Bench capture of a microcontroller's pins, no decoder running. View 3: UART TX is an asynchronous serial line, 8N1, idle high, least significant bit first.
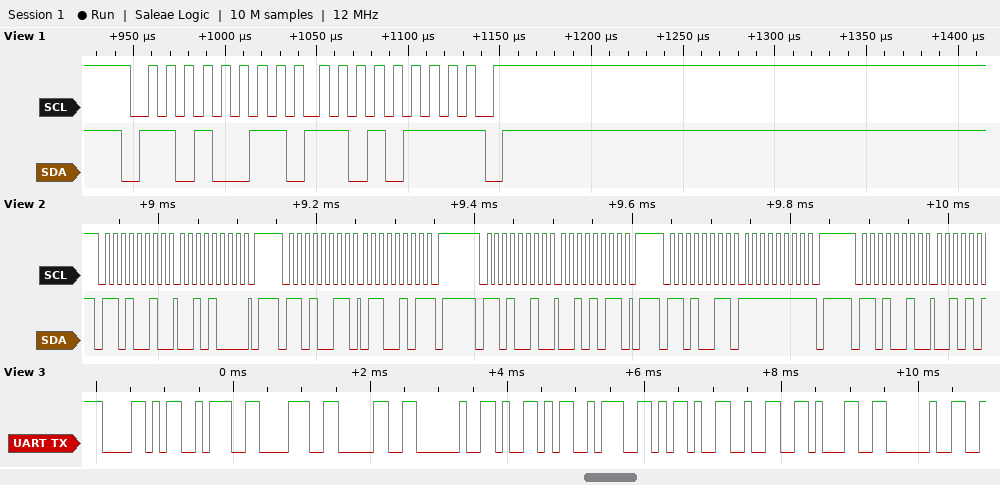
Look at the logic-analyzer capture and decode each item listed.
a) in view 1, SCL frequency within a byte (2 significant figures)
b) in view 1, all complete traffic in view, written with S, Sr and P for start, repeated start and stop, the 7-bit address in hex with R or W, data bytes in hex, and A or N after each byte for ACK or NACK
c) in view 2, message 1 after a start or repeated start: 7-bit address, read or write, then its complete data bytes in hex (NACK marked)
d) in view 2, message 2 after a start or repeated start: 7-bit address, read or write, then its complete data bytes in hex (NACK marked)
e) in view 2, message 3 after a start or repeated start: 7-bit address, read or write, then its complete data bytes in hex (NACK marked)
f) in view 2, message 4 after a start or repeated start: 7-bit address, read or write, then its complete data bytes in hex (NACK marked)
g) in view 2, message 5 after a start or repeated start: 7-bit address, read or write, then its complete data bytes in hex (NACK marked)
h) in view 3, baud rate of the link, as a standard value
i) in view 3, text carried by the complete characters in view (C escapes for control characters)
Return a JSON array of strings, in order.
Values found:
["100 kHz", "S 69R A D7 N P", "0x69 write: 28", "0x69 read: 65 NACK", "0x69 write: 2B", "0x69 read: FF NACK", "0x69 write", "9600 baud", "\"X:80 Y:-21 \""]
